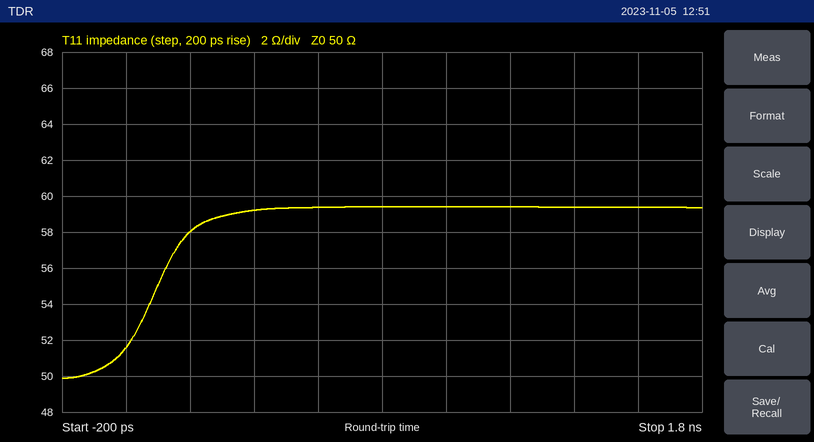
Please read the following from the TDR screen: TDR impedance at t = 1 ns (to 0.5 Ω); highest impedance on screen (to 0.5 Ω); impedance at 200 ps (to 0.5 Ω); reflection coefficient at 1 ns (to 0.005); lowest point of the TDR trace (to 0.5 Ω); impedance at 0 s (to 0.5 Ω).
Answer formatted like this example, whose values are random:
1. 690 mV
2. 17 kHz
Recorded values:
1. 59.5 Ω
2. 59.5 Ω
3. 58.0 Ω
4. +0.085
5. 50.0 Ω
6. 51.5 Ω
